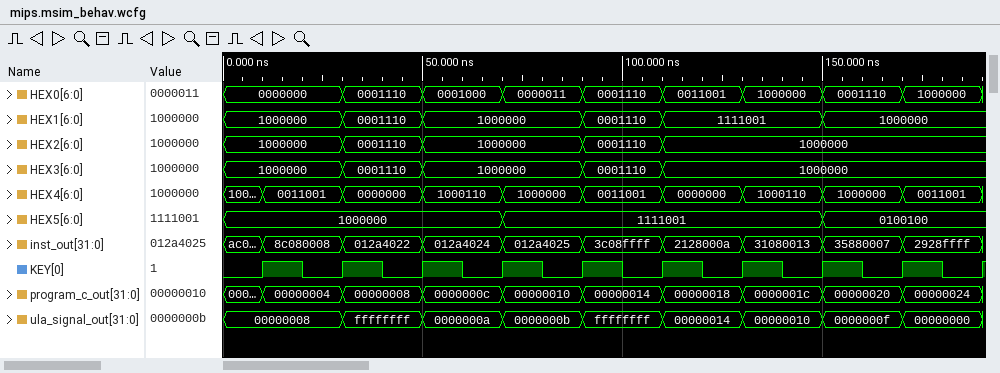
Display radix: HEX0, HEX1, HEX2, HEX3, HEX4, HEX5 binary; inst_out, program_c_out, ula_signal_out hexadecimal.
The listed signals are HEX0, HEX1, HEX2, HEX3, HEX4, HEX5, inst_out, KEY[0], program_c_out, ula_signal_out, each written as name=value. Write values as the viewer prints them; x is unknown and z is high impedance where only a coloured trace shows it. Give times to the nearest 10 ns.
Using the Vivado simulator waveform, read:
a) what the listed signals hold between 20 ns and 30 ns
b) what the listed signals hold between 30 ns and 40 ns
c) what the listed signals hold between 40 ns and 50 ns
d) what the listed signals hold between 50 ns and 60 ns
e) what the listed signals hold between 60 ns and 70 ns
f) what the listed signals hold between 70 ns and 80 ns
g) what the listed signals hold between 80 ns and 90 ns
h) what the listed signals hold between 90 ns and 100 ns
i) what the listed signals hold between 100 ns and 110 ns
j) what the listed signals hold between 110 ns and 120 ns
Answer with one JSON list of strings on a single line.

["HEX0=0000000, HEX1=1000000, HEX2=1000000, HEX3=1000000, HEX4=0011001, HEX5=1000000, inst_out=8c080008, KEY[0]=0, program_c_out=00000004, ula_signal_out=00000008", "HEX0=0001110, HEX1=0001110, HEX2=0001110, HEX3=0001110, HEX4=0000000, HEX5=1000000, inst_out=012a4022, KEY[0]=1, program_c_out=00000008, ula_signal_out=ffffffff", "HEX0=0001110, HEX1=0001110, HEX2=0001110, HEX3=0001110, HEX4=0000000, HEX5=1000000, inst_out=012a4022, KEY[0]=0, program_c_out=00000008, ula_signal_out=ffffffff", "HEX0=0001000, HEX1=1000000, HEX2=1000000, HEX3=1000000, HEX4=1000110, HEX5=1000000, inst_out=012a4024, KEY[0]=1, program_c_out=0000000c, ula_signal_out=0000000a", "HEX0=0001000, HEX1=1000000, HEX2=1000000, HEX3=1000000, HEX4=1000110, HEX5=1000000, inst_out=012a4024, KEY[0]=0, program_c_out=0000000c, ula_signal_out=0000000a", "HEX0=0000011, HEX1=1000000, HEX2=1000000, HEX3=1000000, HEX4=1000000, HEX5=1111001, inst_out=012a4025, KEY[0]=1, program_c_out=00000010, ula_signal_out=0000000b", "HEX0=0000011, HEX1=1000000, HEX2=1000000, HEX3=1000000, HEX4=1000000, HEX5=1111001, inst_out=012a4025, KEY[0]=0, program_c_out=00000010, ula_signal_out=0000000b", "HEX0=0001110, HEX1=0001110, HEX2=0001110, HEX3=0001110, HEX4=0011001, HEX5=1111001, inst_out=3c08ffff, KEY[0]=1, program_c_out=00000014, ula_signal_out=ffffffff", "HEX0=0001110, HEX1=0001110, HEX2=0001110, HEX3=0001110, HEX4=0011001, HEX5=1111001, inst_out=3c08ffff, KEY[0]=0, program_c_out=00000014, ula_signal_out=ffffffff", "HEX0=0011001, HEX1=1111001, HEX2=1000000, HEX3=1000000, HEX4=0000000, HEX5=1111001, inst_out=2128000a, KEY[0]=1, program_c_out=00000018, ula_signal_out=00000014"]
